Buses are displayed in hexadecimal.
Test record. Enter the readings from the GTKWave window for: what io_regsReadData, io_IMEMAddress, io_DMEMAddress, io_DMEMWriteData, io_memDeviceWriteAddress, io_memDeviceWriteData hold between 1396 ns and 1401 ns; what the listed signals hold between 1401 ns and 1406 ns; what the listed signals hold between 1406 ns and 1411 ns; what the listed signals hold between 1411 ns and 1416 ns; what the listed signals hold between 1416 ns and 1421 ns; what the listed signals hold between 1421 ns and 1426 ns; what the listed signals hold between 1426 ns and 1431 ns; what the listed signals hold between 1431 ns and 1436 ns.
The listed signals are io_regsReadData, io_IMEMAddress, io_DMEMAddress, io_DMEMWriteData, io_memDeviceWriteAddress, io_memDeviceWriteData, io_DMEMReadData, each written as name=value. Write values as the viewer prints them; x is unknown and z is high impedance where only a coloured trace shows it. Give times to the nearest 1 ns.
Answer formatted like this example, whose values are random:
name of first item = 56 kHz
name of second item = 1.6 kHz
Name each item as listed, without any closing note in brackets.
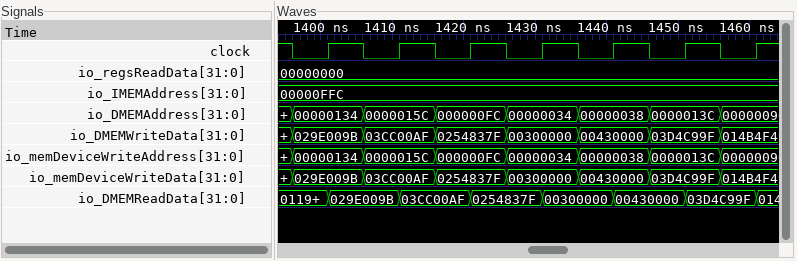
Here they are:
what io_regsReadData, io_IMEMAddress, io_DMEMAddress, io_DMEMWriteData, io_memDeviceWriteAddress, io_memDeviceWriteData hold between 1396 ns and 1401 ns = io_regsReadData=00000000, io_IMEMAddress=00000FFC, io_DMEMAddress=00000134, io_DMEMWriteData=029E009B, io_memDeviceWriteAddress=00000134, io_memDeviceWriteData=029E009B
what the listed signals hold between 1401 ns and 1406 ns = io_regsReadData=00000000, io_IMEMAddress=00000FFC, io_DMEMAddress=00000134, io_DMEMWriteData=029E009B, io_memDeviceWriteAddress=00000134, io_memDeviceWriteData=029E009B, io_DMEMReadData=029E009B
what the listed signals hold between 1406 ns and 1411 ns = io_regsReadData=00000000, io_IMEMAddress=00000FFC, io_DMEMAddress=0000015C, io_DMEMWriteData=03CC00AF, io_memDeviceWriteAddress=0000015C, io_memDeviceWriteData=03CC00AF, io_DMEMReadData=029E009B
what the listed signals hold between 1411 ns and 1416 ns = io_regsReadData=00000000, io_IMEMAddress=00000FFC, io_DMEMAddress=0000015C, io_DMEMWriteData=03CC00AF, io_memDeviceWriteAddress=0000015C, io_memDeviceWriteData=03CC00AF, io_DMEMReadData=03CC00AF
what the listed signals hold between 1416 ns and 1421 ns = io_regsReadData=00000000, io_IMEMAddress=00000FFC, io_DMEMAddress=000000FC, io_DMEMWriteData=0254837F, io_memDeviceWriteAddress=000000FC, io_memDeviceWriteData=0254837F, io_DMEMReadData=03CC00AF
what the listed signals hold between 1421 ns and 1426 ns = io_regsReadData=00000000, io_IMEMAddress=00000FFC, io_DMEMAddress=000000FC, io_DMEMWriteData=0254837F, io_memDeviceWriteAddress=000000FC, io_memDeviceWriteData=0254837F, io_DMEMReadData=0254837F
what the listed signals hold between 1426 ns and 1431 ns = io_regsReadData=00000000, io_IMEMAddress=00000FFC, io_DMEMAddress=00000034, io_DMEMWriteData=00300000, io_memDeviceWriteAddress=00000034, io_memDeviceWriteData=00300000, io_DMEMReadData=0254837F
what the listed signals hold between 1431 ns and 1436 ns = io_regsReadData=00000000, io_IMEMAddress=00000FFC, io_DMEMAddress=00000034, io_DMEMWriteData=00300000, io_memDeviceWriteAddress=00000034, io_memDeviceWriteData=00300000, io_DMEMReadData=00300000
